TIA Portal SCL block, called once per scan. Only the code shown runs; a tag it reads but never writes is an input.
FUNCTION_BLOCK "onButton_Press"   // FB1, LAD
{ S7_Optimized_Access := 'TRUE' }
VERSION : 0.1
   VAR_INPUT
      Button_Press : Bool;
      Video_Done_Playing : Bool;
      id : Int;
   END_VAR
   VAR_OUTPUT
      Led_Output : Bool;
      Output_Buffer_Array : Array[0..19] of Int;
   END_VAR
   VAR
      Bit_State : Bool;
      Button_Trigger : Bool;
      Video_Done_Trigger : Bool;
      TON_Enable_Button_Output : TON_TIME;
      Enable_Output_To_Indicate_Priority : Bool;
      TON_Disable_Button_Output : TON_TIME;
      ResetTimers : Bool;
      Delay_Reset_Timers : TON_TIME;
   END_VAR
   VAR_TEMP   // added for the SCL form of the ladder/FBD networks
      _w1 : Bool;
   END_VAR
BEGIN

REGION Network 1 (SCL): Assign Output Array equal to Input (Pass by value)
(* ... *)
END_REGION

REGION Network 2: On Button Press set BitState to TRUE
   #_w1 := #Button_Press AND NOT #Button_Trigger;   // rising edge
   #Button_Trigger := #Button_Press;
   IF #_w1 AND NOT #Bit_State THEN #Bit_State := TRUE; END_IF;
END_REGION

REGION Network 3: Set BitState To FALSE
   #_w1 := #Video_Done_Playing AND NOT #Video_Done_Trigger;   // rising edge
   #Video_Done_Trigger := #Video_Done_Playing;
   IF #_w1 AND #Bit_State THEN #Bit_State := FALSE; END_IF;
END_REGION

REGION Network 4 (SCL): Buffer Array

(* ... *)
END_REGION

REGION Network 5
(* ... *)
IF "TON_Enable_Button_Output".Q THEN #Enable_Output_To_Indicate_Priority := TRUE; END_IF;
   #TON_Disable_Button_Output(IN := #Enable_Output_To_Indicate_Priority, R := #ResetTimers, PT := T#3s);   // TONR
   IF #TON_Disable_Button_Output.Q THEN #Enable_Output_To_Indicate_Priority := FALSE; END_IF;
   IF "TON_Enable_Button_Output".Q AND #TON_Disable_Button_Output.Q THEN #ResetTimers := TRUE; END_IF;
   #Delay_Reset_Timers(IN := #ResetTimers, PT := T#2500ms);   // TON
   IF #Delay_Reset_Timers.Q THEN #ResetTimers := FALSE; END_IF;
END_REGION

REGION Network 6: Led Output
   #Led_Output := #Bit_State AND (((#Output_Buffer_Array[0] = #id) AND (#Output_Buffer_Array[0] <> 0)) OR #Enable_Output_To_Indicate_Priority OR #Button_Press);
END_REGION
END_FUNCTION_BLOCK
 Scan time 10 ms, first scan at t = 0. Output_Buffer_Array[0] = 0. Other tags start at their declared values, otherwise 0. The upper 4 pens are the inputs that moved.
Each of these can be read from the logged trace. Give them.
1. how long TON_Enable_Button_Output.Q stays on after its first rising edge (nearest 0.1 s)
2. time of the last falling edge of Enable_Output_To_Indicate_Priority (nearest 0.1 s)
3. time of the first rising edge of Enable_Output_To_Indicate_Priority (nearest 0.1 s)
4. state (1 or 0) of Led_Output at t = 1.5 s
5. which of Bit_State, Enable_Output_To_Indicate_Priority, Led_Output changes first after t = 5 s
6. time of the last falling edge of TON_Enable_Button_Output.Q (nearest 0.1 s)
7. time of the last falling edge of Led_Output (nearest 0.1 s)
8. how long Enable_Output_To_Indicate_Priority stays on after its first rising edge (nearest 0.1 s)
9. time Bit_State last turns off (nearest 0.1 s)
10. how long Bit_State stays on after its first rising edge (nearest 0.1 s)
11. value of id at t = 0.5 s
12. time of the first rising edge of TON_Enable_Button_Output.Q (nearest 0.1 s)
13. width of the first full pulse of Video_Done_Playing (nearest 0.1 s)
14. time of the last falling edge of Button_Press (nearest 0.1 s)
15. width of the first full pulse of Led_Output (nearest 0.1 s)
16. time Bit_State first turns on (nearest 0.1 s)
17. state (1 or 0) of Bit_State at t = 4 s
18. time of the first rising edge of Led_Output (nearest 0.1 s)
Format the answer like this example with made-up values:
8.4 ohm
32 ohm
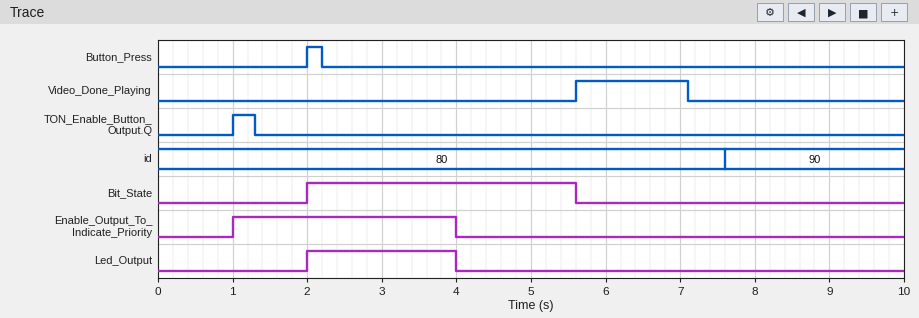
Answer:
0.3 s
4.0 s
1.0 s
0
Bit_State
1.3 s
4.0 s
3.0 s
5.6 s
3.6 s
80
1.0 s
1.5 s
2.2 s
2.0 s
2.0 s
1
2.0 s
